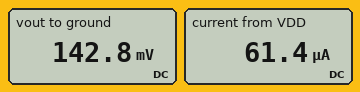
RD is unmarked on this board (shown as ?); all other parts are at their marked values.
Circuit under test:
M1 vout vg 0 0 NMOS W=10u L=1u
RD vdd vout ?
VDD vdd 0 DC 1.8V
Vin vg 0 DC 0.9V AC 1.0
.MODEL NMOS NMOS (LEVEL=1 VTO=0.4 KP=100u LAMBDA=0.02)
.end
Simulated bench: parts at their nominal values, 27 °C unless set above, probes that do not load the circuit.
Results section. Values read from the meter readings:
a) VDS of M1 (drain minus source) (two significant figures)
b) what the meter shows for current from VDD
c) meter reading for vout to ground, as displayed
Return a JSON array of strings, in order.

["140 mV", "61.4 µA", "142.8 mV"]
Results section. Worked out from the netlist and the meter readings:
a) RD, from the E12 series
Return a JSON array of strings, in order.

["27 kΩ"]
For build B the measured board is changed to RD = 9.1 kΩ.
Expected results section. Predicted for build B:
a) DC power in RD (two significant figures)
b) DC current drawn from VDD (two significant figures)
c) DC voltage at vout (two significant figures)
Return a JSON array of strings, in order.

["150 µW", "130 µA", "650 mV"]
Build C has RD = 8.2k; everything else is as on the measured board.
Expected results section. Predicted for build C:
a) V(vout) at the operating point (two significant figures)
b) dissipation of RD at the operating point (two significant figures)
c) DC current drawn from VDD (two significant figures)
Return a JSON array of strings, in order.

["760 mV", "130 µW", "130 µA"]
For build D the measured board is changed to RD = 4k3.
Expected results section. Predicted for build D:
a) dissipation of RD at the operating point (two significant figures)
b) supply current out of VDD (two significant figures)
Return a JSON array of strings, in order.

["71 µW", "130 µA"]
